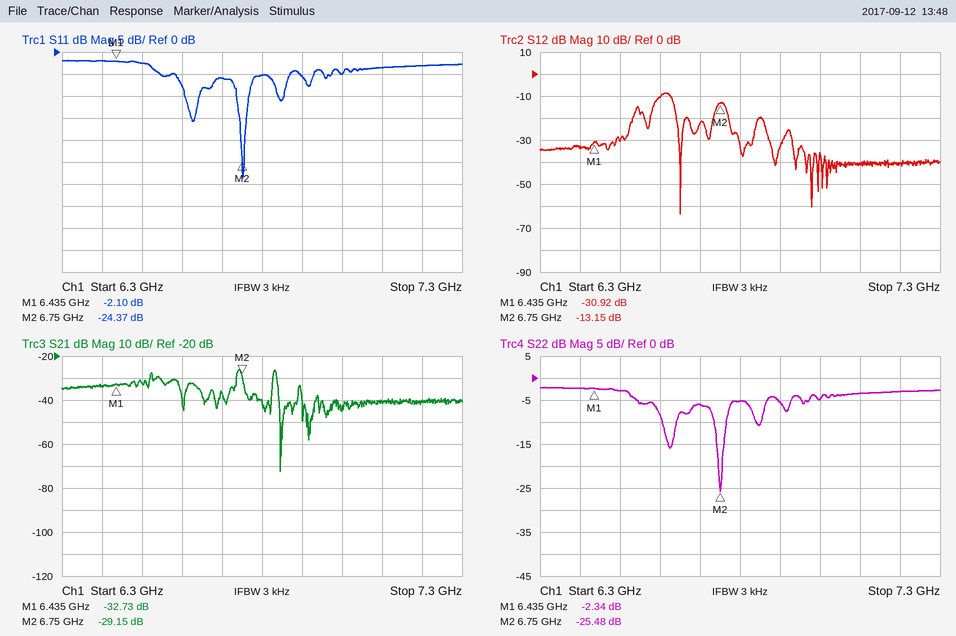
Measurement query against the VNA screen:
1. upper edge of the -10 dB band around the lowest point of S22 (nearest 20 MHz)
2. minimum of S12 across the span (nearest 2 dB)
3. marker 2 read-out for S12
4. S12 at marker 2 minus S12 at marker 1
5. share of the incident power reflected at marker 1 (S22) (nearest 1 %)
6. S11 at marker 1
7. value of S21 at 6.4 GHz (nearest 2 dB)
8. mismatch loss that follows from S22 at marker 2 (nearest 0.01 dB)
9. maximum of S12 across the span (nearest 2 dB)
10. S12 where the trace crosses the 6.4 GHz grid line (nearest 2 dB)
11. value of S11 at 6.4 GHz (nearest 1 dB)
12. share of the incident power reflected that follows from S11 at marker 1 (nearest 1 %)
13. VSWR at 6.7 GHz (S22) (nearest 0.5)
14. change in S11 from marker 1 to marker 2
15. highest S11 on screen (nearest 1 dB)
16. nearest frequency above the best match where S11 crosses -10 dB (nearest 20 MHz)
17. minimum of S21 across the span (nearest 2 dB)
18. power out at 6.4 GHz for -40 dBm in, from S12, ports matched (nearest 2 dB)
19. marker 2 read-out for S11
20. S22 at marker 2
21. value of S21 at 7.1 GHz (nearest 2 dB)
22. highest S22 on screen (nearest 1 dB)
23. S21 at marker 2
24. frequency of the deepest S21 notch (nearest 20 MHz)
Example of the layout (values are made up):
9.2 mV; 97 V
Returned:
6.76 GHz; -64 dB; -13.15 dB; 17.77 dB; 58 %; -2.10 dB; -34 dB; 0.01 dB; -8 dB; -34 dB; -2 dB; 62 %; 3.0; -22.27 dB; -2 dB; 6.76 GHz; -72 dB; -74 dBm; -24.37 dB; -25.48 dB; -40 dB; -2 dB; -29.15 dB; 6.84 GHz
